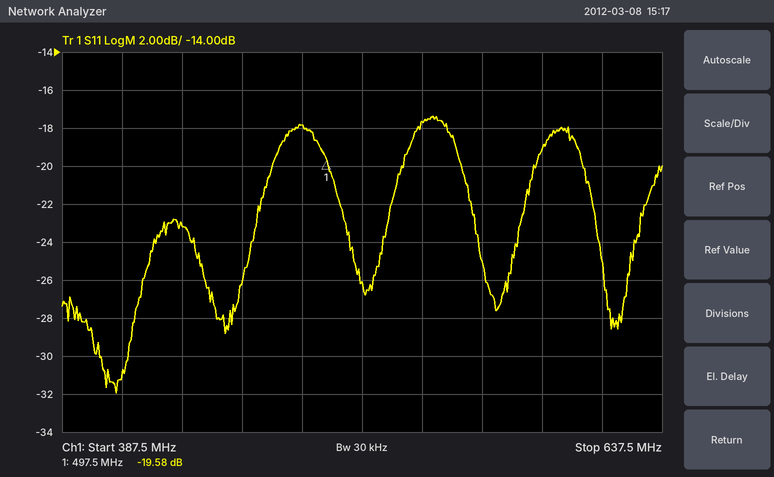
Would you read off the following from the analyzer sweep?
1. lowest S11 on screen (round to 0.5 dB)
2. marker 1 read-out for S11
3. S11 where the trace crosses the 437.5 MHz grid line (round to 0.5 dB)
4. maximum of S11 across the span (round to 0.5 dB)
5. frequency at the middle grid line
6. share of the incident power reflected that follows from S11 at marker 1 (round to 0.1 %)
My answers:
-32.0 dB
-19.58 dB
-23.0 dB
-17.5 dB
512.5 MHz
1.1 %
